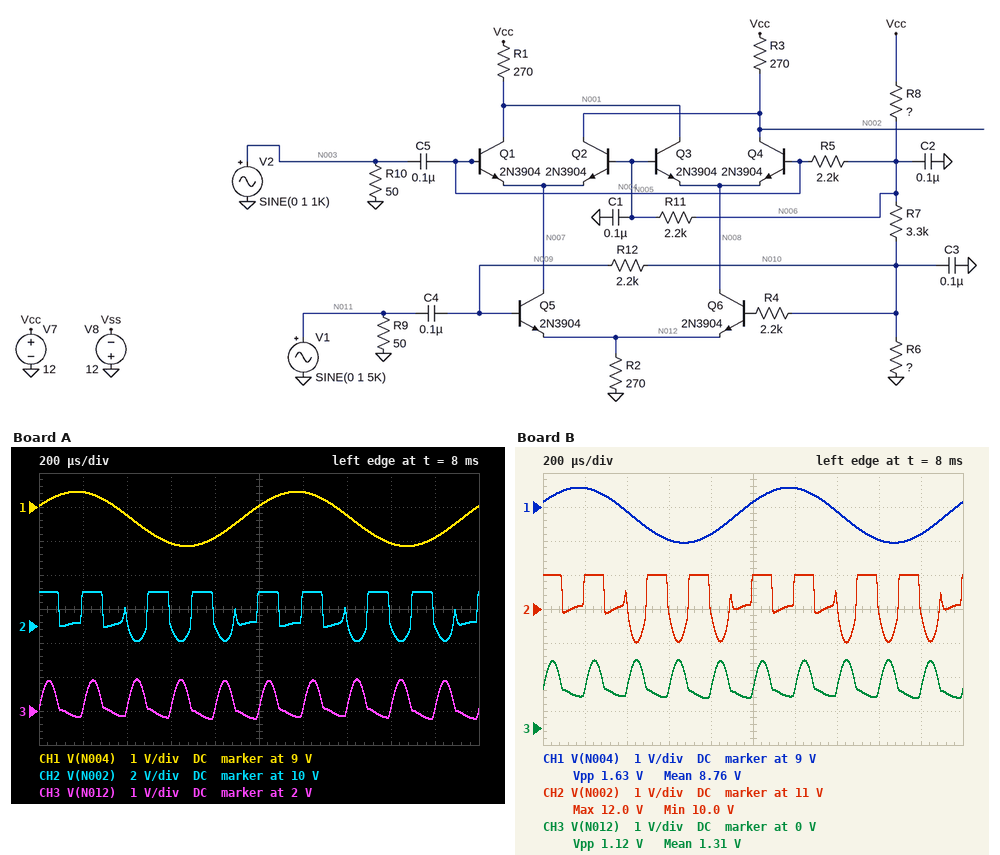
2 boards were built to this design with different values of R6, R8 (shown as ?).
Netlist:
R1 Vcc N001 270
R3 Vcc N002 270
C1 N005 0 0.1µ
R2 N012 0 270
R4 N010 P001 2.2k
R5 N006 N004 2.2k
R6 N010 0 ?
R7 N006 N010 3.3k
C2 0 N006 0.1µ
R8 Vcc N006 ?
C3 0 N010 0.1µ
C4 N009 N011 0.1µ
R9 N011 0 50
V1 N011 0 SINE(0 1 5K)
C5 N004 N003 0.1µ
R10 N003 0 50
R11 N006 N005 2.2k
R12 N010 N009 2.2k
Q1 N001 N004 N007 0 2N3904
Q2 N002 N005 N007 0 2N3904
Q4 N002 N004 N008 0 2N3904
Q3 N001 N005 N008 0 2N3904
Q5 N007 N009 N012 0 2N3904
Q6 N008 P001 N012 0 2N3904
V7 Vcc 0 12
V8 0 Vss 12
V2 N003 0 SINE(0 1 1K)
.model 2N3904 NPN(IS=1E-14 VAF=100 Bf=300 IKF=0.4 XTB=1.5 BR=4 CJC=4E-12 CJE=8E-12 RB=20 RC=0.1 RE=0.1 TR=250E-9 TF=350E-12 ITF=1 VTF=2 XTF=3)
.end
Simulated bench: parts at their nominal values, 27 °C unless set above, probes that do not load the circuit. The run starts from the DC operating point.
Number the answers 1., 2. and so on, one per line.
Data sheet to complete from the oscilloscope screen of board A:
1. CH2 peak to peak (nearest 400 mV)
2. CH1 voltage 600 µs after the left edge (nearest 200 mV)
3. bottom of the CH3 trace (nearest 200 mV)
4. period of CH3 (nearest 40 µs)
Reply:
1. 2.8 V
2. 8.0 V
3. 1.8 V
4. 200 µs
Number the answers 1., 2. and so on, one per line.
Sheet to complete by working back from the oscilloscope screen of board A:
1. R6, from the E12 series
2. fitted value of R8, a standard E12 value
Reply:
1. 1.5 kΩ
2. 1.8 kΩ
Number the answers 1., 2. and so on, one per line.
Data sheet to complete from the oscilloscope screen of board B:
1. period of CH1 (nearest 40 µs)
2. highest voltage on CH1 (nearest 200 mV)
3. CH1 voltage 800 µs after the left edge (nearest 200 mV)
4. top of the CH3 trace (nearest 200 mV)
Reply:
1. 1.00 ms
2. 9.6 V
3. 8.2 V
4. 2.0 V
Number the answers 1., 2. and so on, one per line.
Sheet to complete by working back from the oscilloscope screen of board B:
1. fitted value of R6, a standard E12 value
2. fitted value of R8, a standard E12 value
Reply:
1. 820 Ω
2. 1.5 kΩ
